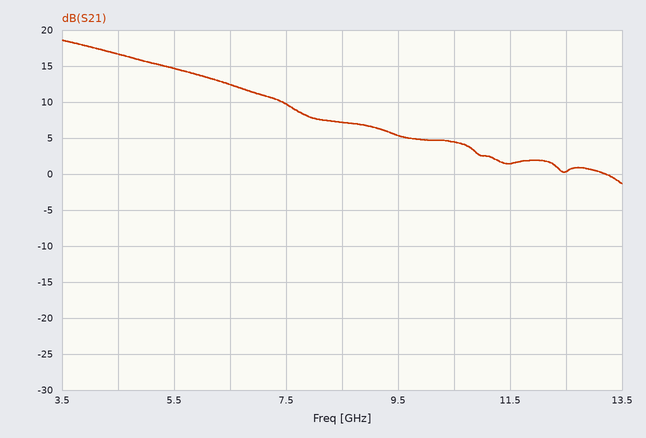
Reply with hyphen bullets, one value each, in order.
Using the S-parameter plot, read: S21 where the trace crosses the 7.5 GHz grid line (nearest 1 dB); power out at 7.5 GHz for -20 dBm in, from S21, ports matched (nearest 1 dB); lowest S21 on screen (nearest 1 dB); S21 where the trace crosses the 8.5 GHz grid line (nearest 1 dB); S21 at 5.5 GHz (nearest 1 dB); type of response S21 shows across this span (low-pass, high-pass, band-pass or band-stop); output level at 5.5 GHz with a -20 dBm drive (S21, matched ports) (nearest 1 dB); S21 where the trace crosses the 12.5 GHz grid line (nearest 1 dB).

- 10 dB
- -10 dBm
- -1 dB
- 7 dB
- 15 dB
- low-pass
- -5 dBm
- 0 dB
